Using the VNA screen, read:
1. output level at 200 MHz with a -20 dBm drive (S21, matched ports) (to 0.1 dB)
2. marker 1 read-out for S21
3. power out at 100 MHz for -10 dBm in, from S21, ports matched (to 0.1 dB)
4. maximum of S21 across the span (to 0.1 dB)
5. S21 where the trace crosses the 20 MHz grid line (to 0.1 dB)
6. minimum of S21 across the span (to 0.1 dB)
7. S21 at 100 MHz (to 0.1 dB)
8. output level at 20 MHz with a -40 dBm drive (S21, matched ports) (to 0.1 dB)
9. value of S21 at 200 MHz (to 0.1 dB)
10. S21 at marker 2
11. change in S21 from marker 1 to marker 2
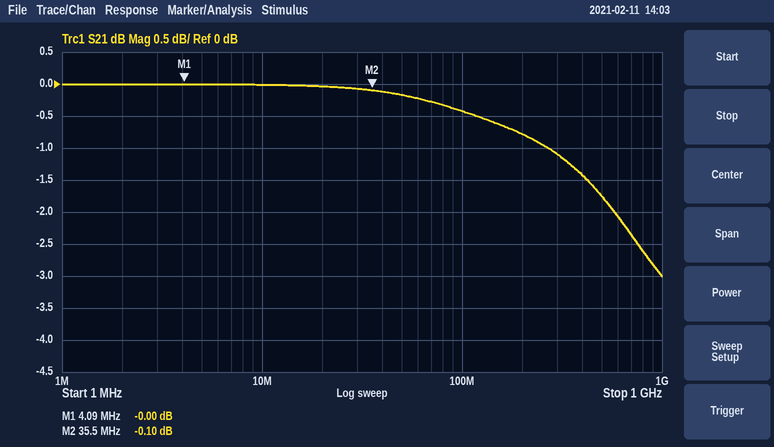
-20.8 dBm
-0.00 dB
-10.4 dBm
0.0 dB
0.0 dB
-3.0 dB
-0.4 dB
-40.0 dBm
-0.8 dB
-0.10 dB
-0.10 dB
